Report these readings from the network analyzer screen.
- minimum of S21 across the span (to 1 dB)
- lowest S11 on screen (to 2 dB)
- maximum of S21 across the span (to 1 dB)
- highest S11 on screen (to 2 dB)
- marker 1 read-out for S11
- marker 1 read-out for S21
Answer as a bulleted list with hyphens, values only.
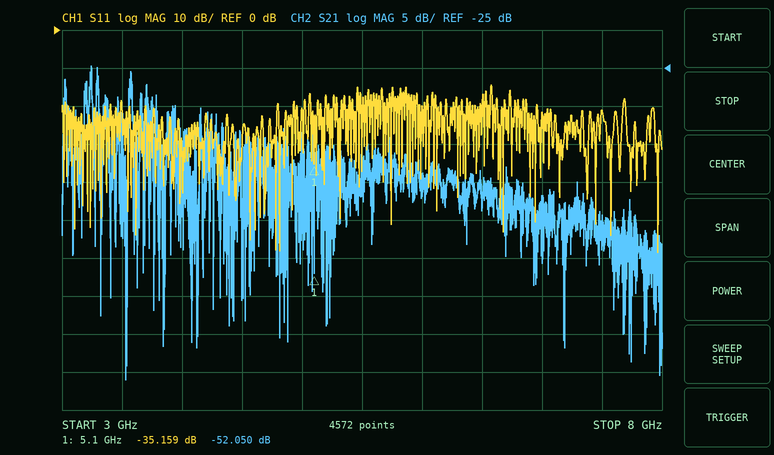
- -66 dB
- -58 dB
- -25 dB
- -14 dB
- -35.159 dB
- -52.050 dB
